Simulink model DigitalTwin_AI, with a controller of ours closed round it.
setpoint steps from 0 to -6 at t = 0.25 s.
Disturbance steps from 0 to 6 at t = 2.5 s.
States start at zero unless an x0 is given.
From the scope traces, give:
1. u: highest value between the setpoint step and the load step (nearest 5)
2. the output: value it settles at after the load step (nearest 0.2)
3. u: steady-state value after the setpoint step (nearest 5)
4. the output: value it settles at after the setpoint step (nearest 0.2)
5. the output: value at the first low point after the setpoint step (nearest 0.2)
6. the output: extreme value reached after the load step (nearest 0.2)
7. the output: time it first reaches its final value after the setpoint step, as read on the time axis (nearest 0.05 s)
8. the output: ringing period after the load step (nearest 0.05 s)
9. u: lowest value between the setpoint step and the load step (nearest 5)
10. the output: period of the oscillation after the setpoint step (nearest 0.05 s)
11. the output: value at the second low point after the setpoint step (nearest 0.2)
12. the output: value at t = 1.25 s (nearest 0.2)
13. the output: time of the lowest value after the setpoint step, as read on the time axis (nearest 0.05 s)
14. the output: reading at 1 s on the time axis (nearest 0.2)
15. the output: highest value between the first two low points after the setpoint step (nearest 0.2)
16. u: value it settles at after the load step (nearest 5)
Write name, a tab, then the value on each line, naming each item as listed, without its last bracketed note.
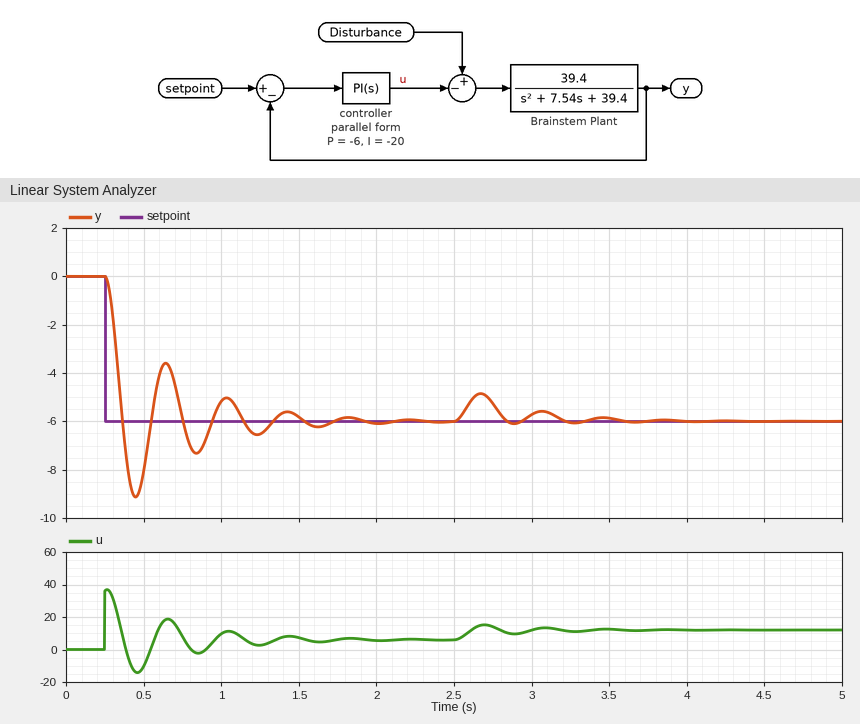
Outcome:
u: highest value between the setpoint step and the load step	35
the output: value it settles at after the load step	-6.0
u: steady-state value after the setpoint step	5
the output: value it settles at after the setpoint step	-6.0
the output: value at the first low point after the setpoint step	-9.2
the output: extreme value reached after the load step	-4.8
the output: time it first reaches its final value after the setpoint step, as read on the time axis	0.35 s
the output: ringing period after the load step	0.40 s
u: lowest value between the setpoint step and the load step	-15
the output: period of the oscillation after the setpoint step	0.40 s
the output: value at the second low point after the setpoint step	-7.4
the output: value at t = 1.25 s	-6.6
the output: time of the lowest value after the setpoint step, as read on the time axis	0.45 s
the output: reading at 1 s on the time axis	-5.2
the output: highest value between the first two low points after the setpoint step	-3.6
u: value it settles at after the load step	10
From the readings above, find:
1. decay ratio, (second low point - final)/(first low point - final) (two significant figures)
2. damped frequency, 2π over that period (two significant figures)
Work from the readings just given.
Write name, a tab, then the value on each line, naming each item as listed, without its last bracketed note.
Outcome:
decay ratio, (second low point - final)/(first low point - final)	0.44
damped frequency, 2π over that period	16 rad/s
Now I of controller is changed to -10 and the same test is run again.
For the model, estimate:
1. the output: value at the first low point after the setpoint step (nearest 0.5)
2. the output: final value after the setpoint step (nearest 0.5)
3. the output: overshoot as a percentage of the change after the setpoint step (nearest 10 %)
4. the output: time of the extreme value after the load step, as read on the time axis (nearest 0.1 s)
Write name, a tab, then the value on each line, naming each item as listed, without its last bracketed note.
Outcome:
the output: value at the first low point after the setpoint step	-8.5
the output: final value after the setpoint step	-6.0
the output: overshoot as a percentage of the change after the setpoint step	40 %
the output: time of the extreme value after the load step, as read on the time axis	2.7 s
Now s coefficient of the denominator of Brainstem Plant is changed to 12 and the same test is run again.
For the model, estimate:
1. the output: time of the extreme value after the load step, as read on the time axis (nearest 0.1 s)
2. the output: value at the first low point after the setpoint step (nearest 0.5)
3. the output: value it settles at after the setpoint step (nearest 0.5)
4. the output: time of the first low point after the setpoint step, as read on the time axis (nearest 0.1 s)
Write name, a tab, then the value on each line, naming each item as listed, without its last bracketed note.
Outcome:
the output: time of the extreme value after the load step, as read on the time axis	2.7 s
the output: value at the first low point after the setpoint step	-8.0
the output: value it settles at after the setpoint step	-6.0
the output: time of the first low point after the setpoint step, as read on the time axis	0.5 s
